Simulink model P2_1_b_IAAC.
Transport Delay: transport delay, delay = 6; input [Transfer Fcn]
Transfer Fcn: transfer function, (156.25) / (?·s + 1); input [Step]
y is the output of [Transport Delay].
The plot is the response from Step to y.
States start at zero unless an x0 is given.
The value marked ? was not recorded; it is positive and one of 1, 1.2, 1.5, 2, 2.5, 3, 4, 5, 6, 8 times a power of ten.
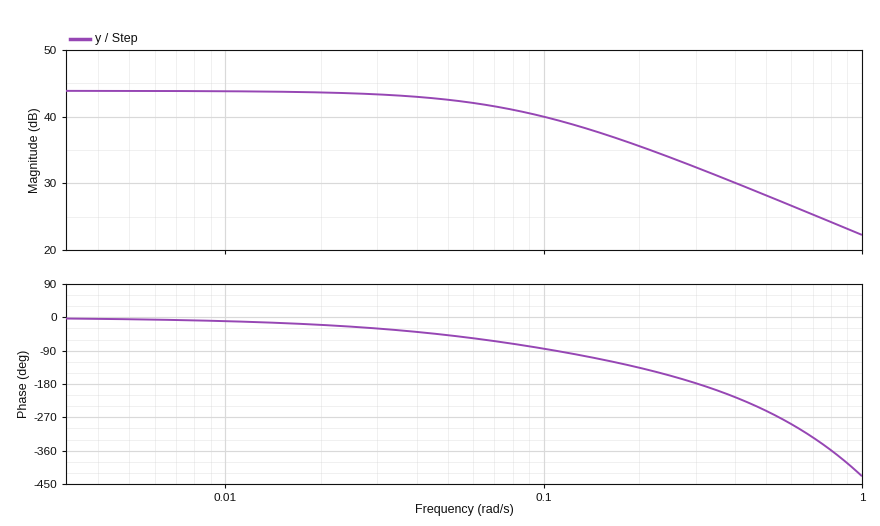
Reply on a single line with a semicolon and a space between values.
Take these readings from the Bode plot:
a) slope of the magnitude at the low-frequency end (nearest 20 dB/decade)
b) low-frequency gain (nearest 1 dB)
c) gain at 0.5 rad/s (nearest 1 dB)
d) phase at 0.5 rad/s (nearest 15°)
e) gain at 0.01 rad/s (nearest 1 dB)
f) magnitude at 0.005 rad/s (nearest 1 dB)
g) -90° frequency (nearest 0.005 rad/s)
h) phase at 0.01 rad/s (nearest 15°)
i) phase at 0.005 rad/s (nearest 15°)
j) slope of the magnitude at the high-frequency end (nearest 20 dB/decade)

0 dB/decade; 44 dB; 28 dB; -255°; 44 dB; 44 dB; 0.110 rad/s; -15°; 0°; -20 dB/decade
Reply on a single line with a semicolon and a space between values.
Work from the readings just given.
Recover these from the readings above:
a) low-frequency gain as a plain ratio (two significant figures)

160
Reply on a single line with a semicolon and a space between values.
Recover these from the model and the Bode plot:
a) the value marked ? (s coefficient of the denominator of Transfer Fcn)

12
